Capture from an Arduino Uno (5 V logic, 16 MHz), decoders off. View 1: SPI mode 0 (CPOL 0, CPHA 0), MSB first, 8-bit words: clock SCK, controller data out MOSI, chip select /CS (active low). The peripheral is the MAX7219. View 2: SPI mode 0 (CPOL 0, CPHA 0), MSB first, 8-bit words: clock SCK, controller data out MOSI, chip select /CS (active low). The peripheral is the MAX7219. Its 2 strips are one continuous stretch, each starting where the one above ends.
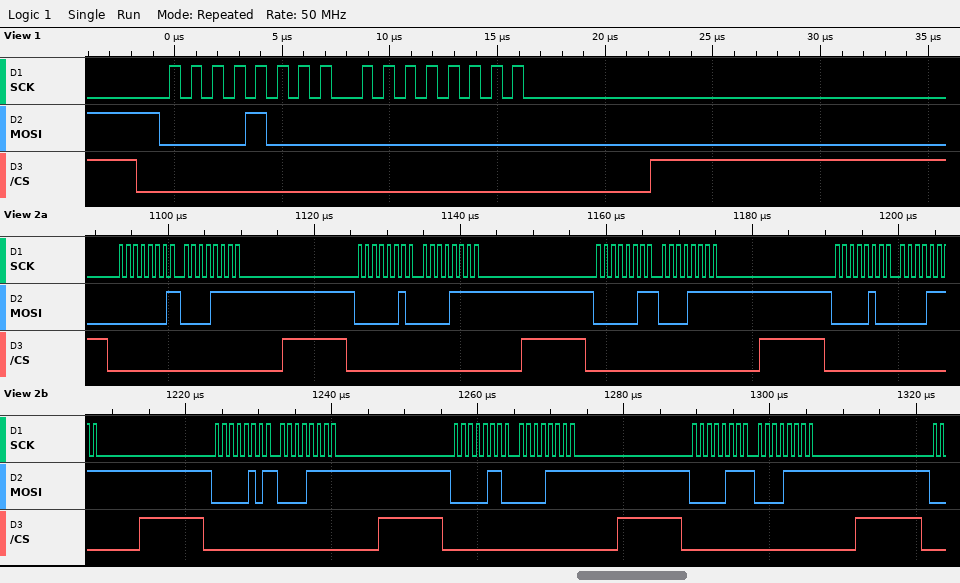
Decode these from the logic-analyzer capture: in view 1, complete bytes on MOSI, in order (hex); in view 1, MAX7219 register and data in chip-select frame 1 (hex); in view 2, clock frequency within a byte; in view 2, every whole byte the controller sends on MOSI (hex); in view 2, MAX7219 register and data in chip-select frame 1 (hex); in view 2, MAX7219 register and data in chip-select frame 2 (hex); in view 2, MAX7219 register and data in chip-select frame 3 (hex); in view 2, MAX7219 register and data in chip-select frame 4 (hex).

08 00
register 0x8, data 0x00
1 MHz
0x01 0x0F 0x02 0x0F 0x03 0x0F 0x04 0x0F 0x05 0x0F 0x06 0x0F 0x07 0x0F
register 0x1, data 0x0F
register 0x2, data 0x0F
register 0x3, data 0x0F
register 0x4, data 0x0F
